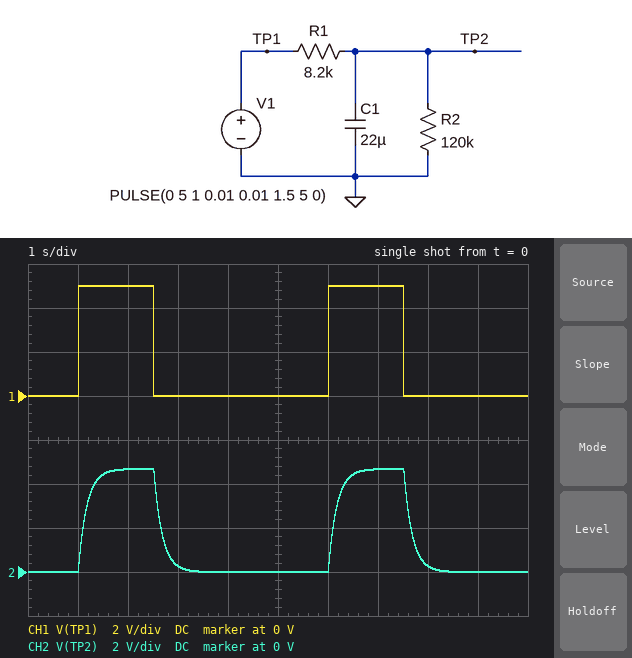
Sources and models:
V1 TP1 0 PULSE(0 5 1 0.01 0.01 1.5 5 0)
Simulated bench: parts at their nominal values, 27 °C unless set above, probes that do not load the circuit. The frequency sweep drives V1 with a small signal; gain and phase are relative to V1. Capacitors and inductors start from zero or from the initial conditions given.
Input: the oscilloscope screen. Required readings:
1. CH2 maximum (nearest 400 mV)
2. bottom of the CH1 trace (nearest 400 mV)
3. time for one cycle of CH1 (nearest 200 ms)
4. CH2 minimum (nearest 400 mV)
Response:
4.8 V
0 V
5.0 s
0 V
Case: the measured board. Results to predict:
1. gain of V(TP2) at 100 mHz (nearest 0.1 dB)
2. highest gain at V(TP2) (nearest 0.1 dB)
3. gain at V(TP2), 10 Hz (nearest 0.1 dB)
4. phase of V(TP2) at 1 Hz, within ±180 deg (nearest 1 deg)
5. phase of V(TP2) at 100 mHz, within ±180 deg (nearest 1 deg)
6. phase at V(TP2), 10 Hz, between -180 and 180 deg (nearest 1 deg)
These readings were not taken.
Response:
-0.6 dB
-0.6 dB
-21.1 dB
-47 deg
-6 deg
-85 deg
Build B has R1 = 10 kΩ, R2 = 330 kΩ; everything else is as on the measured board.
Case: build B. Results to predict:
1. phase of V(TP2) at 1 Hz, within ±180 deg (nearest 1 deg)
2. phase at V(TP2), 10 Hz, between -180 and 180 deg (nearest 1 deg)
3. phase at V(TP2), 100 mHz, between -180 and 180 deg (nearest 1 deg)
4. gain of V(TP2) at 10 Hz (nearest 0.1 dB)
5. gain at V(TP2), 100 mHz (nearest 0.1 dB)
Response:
-53 deg
-86 deg
-8 deg
-22.8 dB
-0.3 dB
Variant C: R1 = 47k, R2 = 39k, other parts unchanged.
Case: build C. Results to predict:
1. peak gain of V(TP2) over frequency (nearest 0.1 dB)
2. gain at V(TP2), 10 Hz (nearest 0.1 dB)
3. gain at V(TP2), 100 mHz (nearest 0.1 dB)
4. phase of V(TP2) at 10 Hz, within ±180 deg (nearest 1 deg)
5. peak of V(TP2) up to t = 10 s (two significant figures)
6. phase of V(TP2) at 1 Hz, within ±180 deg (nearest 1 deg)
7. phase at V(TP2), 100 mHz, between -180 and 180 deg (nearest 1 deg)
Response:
-6.9 dB
-36.3 dB
-7.2 dB
-88 deg
2.2 V
-71 deg
-16 deg
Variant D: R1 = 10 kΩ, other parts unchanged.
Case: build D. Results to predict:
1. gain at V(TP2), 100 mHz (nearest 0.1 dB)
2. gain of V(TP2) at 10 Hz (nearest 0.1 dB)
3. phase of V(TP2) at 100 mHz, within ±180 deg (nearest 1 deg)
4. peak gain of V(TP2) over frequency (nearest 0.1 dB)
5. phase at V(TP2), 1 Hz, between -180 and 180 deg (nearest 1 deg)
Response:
-0.8 dB
-22.8 dB
-7 deg
-0.7 dB
-52 deg
